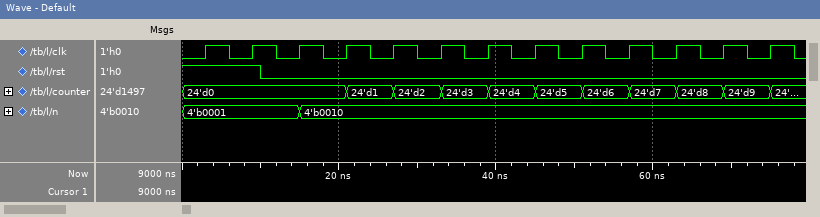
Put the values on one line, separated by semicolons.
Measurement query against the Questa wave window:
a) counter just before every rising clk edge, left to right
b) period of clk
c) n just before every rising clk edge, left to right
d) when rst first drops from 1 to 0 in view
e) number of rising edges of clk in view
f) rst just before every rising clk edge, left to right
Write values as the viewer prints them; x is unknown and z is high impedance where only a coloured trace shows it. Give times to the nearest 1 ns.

24'd0, 24'd0, 24'd0, 24'd0, 24'd1, 24'd2, 24'd3, 24'd4, 24'd5, 24'd6, 24'd7, 24'd8, 24'd9; 6 ns; 4'b0001, 4'b0001, 4'b0001, 4'b0010, 4'b0010, 4'b0010, 4'b0010, 4'b0010, 4'b0010, 4'b0010, 4'b0010, 4'b0010, 4'b0010; 10 ns; 13; 1 1 0 0 0 0 0 0 0 0 0 0 0
